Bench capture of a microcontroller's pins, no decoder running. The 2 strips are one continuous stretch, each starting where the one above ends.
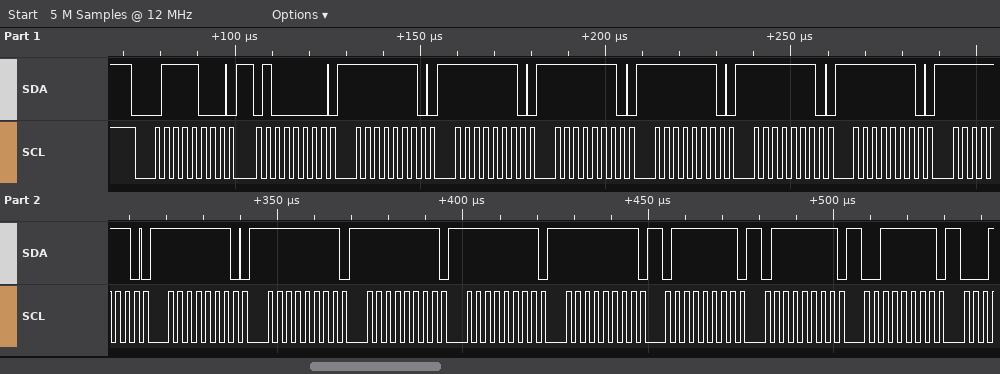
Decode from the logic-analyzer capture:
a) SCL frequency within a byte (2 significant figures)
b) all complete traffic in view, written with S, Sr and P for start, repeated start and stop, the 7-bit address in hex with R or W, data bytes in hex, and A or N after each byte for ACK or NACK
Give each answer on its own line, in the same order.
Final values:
400 kHz
S 3CW A 40 A FE A FE A FE A FE A FE A FE A FE A FE A FF A FF A FF A FF A 7F A 7F A 3F A
